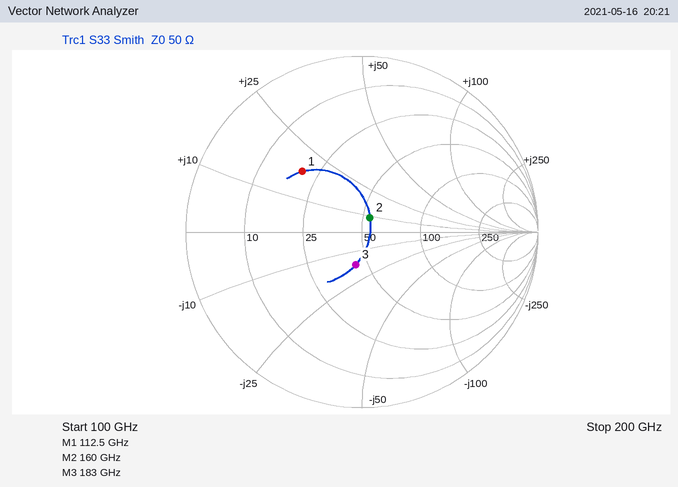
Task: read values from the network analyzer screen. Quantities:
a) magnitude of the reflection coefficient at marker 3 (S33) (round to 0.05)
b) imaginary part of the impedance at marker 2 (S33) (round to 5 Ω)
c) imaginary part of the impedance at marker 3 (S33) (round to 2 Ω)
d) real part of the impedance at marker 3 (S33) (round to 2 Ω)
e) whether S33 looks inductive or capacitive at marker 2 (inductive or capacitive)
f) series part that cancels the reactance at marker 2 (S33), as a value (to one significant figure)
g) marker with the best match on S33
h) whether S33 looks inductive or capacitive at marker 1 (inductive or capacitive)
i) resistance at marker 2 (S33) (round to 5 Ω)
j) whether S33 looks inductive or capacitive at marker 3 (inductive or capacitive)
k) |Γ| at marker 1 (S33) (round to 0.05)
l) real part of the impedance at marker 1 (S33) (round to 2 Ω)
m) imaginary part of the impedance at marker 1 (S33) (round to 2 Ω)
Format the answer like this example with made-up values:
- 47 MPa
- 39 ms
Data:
- 0.20
- +10 Ω
- -16 Ω
- 44 Ω
- inductive
- 100 fF
- marker 2
- inductive
- 55 Ω
- capacitive
- 0.50
- 20 Ω
- +18 Ω
